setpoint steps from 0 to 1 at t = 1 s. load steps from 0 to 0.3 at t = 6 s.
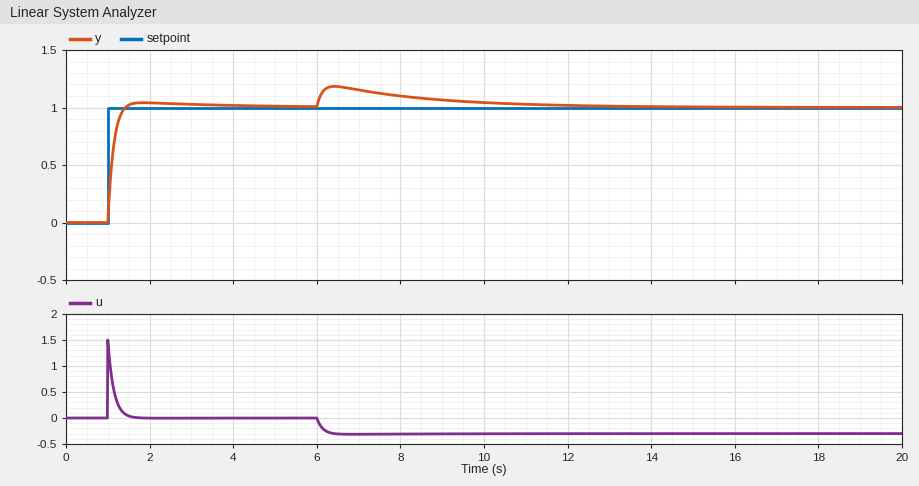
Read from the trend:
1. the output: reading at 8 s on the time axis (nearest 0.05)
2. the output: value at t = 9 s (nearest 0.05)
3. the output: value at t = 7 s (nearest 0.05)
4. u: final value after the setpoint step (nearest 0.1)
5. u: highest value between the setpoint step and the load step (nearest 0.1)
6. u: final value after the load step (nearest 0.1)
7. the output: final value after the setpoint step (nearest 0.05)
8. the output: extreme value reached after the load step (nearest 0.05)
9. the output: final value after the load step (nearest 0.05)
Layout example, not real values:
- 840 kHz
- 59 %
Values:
- 1.10
- 1.05
- 1.15
- 0.0
- 1.5
- -0.3
- 1.00
- 1.20
- 1.00
